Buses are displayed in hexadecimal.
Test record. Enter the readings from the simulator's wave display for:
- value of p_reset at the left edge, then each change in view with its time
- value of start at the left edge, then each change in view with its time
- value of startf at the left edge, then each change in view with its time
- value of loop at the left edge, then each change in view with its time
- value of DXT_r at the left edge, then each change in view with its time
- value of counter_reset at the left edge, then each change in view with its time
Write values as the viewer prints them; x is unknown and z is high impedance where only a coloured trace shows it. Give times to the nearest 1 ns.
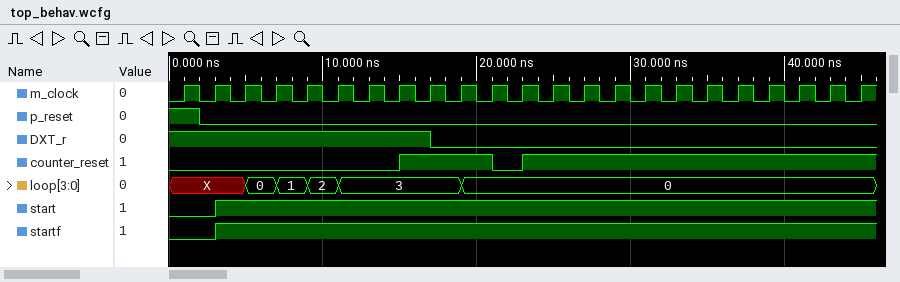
1, 0 at 2 ns
0, 1 at 3 ns
0, 1 at 3 ns
X, 0 at 5 ns, 1 at 7 ns, 2 at 9 ns, 3 at 11 ns, 0 at 19 ns
1, 0 at 17 ns
0, 1 at 15 ns, 0 at 21 ns, 1 at 23 ns
